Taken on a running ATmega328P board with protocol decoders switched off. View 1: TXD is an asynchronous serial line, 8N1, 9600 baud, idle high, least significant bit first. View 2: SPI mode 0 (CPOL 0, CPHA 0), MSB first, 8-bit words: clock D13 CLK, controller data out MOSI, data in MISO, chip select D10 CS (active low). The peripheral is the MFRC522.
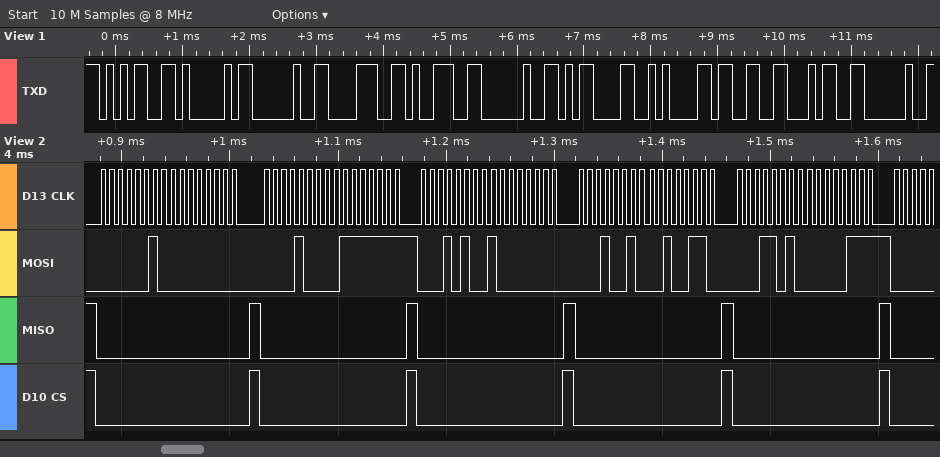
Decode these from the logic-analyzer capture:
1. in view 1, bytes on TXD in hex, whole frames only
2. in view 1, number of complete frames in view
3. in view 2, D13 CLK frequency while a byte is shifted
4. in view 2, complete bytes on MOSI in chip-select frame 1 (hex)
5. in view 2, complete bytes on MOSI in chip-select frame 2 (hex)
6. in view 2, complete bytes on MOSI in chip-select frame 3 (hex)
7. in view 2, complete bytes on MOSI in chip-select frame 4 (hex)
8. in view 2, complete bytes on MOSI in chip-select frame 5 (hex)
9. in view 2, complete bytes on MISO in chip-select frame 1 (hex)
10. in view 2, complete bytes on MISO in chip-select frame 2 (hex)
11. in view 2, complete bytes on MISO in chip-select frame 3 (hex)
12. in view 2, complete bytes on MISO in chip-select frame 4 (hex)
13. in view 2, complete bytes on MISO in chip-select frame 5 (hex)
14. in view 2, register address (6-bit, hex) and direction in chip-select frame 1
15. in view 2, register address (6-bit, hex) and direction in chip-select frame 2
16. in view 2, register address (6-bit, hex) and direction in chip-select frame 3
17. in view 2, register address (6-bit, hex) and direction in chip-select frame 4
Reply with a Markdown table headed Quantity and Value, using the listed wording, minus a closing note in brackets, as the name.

| Quantity | Value |
|---|---|
| in view 1, bytes on TXD in hex, whole frames only | 35 41 20 38 39 20 0D 0A 33 34 20 |
| in view 1, number of complete frames in view | 11 |
| in view 2, D13 CLK frequency while a byte is shifted | 125 kHz |
| in view 2, complete bytes on MOSI in chip-select frame 1 | 02 00 |
| in view 2, complete bytes on MOSI in chip-select frame 2 | 08 7F |
| in view 2, complete bytes on MOSI in chip-select frame 3 | 14 80 |
| in view 2, complete bytes on MOSI in chip-select frame 4 | 12 26 |
| in view 2, complete bytes on MOSI in chip-select frame 5 | 1A 07 |
| in view 2, complete bytes on MISO in chip-select frame 1 | 00 00 |
| in view 2, complete bytes on MISO in chip-select frame 2 | 00 00 |
| in view 2, complete bytes on MISO in chip-select frame 3 | 00 00 |
| in view 2, complete bytes on MISO in chip-select frame 4 | 00 00 |
| in view 2, complete bytes on MISO in chip-select frame 5 | 00 00 |
| in view 2, register address (6-bit, hex) and direction in chip-select frame 1 | 0x01 write |
| in view 2, register address (6-bit, hex) and direction in chip-select frame 2 | 0x04 write |
| in view 2, register address (6-bit, hex) and direction in chip-select frame 3 | 0x0A write |
| in view 2, register address (6-bit, hex) and direction in chip-select frame 4 | 0x09 write |
